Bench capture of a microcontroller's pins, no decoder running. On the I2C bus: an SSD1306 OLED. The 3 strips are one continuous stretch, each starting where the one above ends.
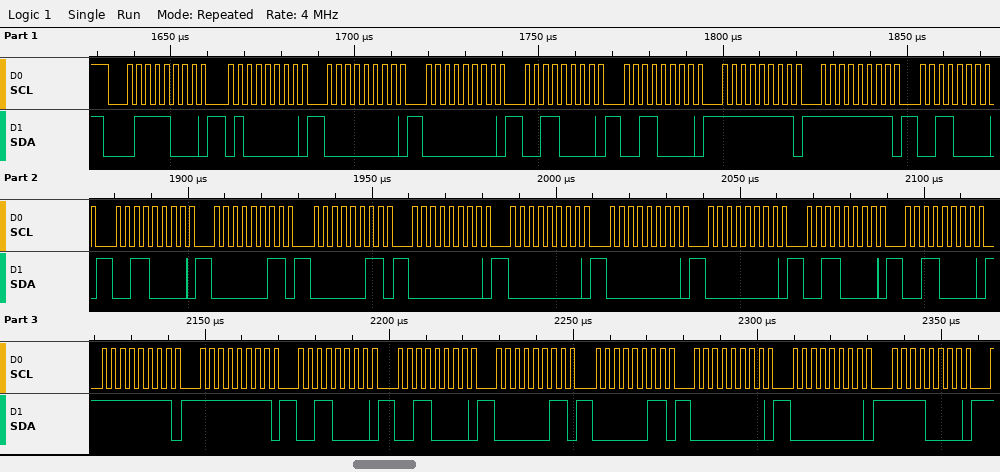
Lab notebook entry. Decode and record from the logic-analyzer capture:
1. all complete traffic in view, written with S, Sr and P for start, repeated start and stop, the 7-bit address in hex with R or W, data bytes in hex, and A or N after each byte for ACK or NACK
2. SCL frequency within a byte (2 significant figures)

S 3CW A 40 A 00 A 00 A 30 A 30 A FF A FF A 30 A 30 A 03 A 03 A 00 A 00 A 00 A 00 A 30 A 30 A FF A FF A 30 A 30 A 03 A 03 A 00 A 00 A F0 A
400 kHz
